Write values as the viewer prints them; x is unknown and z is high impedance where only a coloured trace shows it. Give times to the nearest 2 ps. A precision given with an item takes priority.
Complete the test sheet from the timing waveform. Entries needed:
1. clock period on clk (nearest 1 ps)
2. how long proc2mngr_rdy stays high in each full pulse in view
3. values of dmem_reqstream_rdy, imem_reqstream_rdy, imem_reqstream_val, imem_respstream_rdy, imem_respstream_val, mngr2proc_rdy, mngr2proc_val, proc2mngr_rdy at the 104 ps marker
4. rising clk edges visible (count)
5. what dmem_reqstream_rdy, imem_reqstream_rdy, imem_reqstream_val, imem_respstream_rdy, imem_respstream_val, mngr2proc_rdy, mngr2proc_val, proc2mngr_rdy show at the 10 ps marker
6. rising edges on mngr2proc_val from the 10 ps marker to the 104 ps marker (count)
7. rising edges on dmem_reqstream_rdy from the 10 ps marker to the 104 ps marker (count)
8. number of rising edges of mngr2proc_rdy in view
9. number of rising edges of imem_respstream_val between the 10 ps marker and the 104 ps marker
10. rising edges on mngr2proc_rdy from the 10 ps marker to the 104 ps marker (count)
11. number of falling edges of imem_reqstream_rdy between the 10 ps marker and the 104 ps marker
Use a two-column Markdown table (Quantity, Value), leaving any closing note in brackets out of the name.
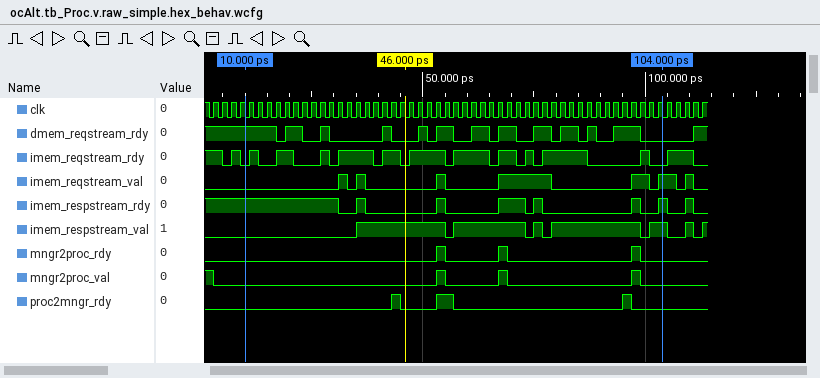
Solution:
| Quantity | Value |
|---|---|
| clock period on clk | 2 ps |
| how long proc2mngr_rdy stays high in each full pulse in view | 2 ps, 4 ps, 2 ps |
| values of dmem_reqstream_rdy, imem_reqstream_rdy, imem_reqstream_val, imem_respstream_rdy, imem_respstream_val, mngr2proc_rdy, mngr2proc_val, proc2mngr_rdy at the 104 ps marker | dmem_reqstream_rdy=0, imem_reqstream_rdy=0, imem_reqstream_val=1, imem_respstream_rdy=1, imem_respstream_val=1, mngr2proc_rdy=0, mngr2proc_val=0, proc2mngr_rdy=0 |
| rising clk edges visible | 56 |
| what dmem_reqstream_rdy, imem_reqstream_rdy, imem_reqstream_val, imem_respstream_rdy, imem_respstream_val, mngr2proc_rdy, mngr2proc_val, proc2mngr_rdy show at the 10 ps marker | dmem_reqstream_rdy=1, imem_reqstream_rdy=0, imem_reqstream_val=0, imem_respstream_rdy=1, imem_respstream_val=0, mngr2proc_rdy=0, mngr2proc_val=0, proc2mngr_rdy=0 |
| rising edges on mngr2proc_val from the 10 ps marker to the 104 ps marker | 3 |
| rising edges on dmem_reqstream_rdy from the 10 ps marker to the 104 ps marker | 11 |
| number of rising edges of mngr2proc_rdy in view | 3 |
| number of rising edges of imem_respstream_val between the 10 ps marker and the 104 ps marker | 5 |
| rising edges on mngr2proc_rdy from the 10 ps marker to the 104 ps marker | 3 |
| number of falling edges of imem_reqstream_rdy between the 10 ps marker and the 104 ps marker | 11 |
